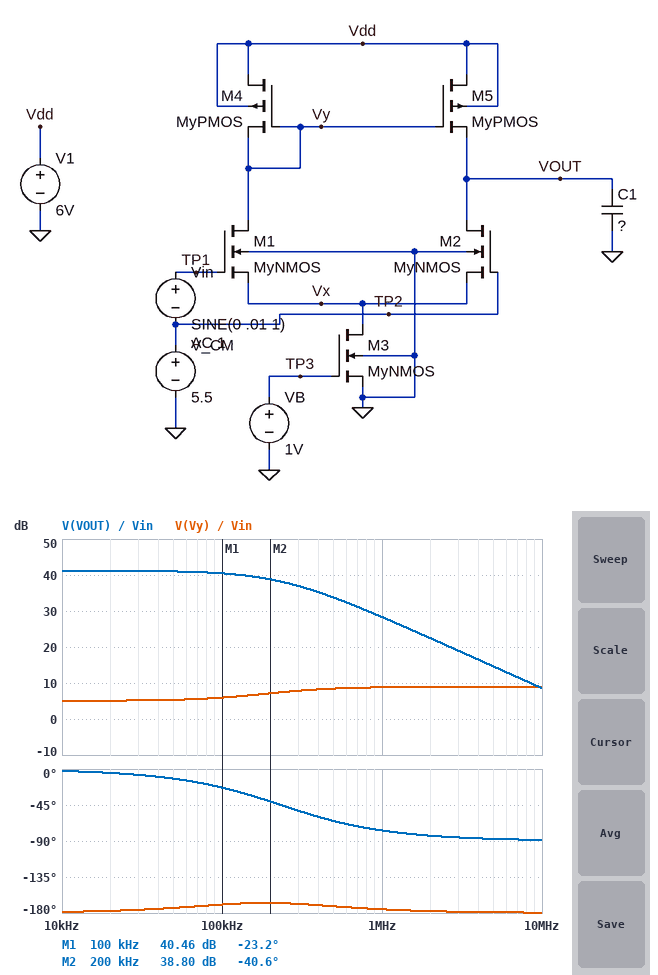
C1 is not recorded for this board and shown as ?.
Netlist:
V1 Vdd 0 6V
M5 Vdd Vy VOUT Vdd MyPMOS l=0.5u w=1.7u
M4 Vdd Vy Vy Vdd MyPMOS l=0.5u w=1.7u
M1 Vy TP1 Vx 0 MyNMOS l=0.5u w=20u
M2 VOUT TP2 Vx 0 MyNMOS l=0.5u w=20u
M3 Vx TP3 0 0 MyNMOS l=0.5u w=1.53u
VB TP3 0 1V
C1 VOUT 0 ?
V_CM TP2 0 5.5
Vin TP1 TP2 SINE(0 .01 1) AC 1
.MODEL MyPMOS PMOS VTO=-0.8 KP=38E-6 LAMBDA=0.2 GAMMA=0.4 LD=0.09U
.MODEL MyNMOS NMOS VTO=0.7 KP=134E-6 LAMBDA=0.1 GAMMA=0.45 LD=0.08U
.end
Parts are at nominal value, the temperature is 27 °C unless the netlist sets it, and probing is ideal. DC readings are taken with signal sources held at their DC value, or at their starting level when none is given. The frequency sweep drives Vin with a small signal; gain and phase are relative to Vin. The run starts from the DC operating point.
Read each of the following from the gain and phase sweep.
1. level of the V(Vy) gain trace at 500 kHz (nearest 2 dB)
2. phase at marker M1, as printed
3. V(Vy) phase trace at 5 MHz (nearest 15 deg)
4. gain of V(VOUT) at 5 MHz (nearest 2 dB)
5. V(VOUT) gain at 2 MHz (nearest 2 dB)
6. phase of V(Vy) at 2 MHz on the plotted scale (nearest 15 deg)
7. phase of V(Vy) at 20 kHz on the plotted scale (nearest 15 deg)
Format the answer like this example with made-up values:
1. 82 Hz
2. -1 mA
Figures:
1. 8 dB
2. -23.2 deg
3. -180 deg
4. 14 dB
5. 22 dB
6. -180 deg
7. -180 deg
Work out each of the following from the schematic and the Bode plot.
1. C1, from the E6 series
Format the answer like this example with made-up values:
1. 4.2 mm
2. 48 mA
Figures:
1. 3.3 pF
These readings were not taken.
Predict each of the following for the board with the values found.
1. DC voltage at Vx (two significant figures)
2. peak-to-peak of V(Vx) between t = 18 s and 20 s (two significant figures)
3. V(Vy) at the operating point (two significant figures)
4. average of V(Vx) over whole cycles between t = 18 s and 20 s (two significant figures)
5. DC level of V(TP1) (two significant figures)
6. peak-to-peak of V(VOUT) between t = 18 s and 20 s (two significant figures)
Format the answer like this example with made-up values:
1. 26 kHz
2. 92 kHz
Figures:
1. 4.1 V
2. 13 mV
3. 4.8 V
4. 4.1 V
5. 5.5 V
6. 1.5 V
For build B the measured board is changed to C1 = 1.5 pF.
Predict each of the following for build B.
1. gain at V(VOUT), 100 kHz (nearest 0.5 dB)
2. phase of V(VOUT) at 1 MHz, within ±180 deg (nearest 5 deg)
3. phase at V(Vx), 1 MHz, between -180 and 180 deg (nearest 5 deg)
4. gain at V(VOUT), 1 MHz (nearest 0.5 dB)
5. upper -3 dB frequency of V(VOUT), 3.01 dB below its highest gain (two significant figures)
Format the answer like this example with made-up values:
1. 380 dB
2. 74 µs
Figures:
1. 41.0 dB
2. -65 deg
3. -10 deg
4. 34.5 dB
5. 510 kHz
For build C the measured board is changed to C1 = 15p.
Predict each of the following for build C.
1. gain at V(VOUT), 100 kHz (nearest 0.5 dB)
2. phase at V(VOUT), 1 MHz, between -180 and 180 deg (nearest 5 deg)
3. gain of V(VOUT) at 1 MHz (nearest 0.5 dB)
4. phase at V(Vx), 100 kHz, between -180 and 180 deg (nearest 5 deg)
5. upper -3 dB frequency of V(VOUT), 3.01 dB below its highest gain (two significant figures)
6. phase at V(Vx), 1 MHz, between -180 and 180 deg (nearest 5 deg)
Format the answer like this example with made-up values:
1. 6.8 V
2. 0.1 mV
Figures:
1. 34.5 dB
2. -85 deg
3. 15.5 dB
4. -10 deg
5. 51 kHz
6. 0 deg
